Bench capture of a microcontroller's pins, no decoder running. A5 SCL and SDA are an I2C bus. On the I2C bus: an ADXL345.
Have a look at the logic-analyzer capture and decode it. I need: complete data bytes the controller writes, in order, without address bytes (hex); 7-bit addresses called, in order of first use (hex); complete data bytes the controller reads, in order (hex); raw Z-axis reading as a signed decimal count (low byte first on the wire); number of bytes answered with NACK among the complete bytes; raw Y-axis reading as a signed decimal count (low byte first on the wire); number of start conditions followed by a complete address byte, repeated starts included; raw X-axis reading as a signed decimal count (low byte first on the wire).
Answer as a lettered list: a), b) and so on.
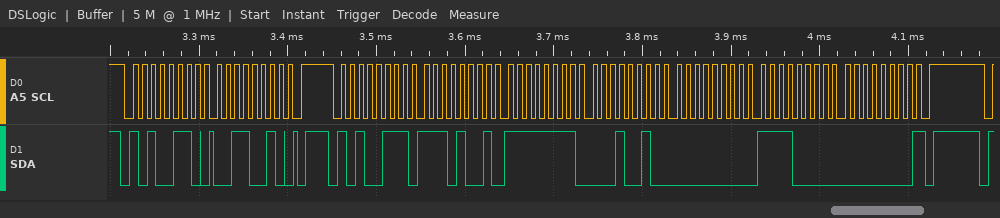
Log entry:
a) 32
b) 0x53
c) E9 FF 12 00 F0 00
d) 240
e) 1
f) 18
g) 2
h) -23
